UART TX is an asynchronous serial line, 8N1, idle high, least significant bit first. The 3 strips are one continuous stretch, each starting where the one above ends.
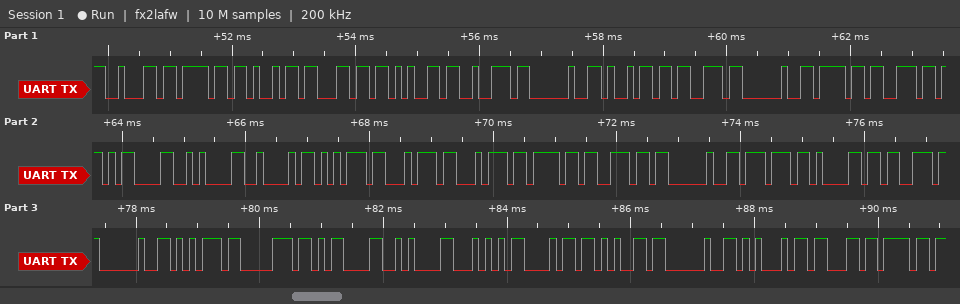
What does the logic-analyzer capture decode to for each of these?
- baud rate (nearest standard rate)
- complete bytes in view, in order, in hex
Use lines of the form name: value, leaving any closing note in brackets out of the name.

baud rate: 9600 baud
complete bytes in view, in order, in hex: 62 6F 69 6C 65 72 20 69 73 20 6F 6E 0D 0A 42 75 74 74 6F 6E 20 77 61 73 20 75 70 0D 0A 54 68 65 20 45 63 6F
